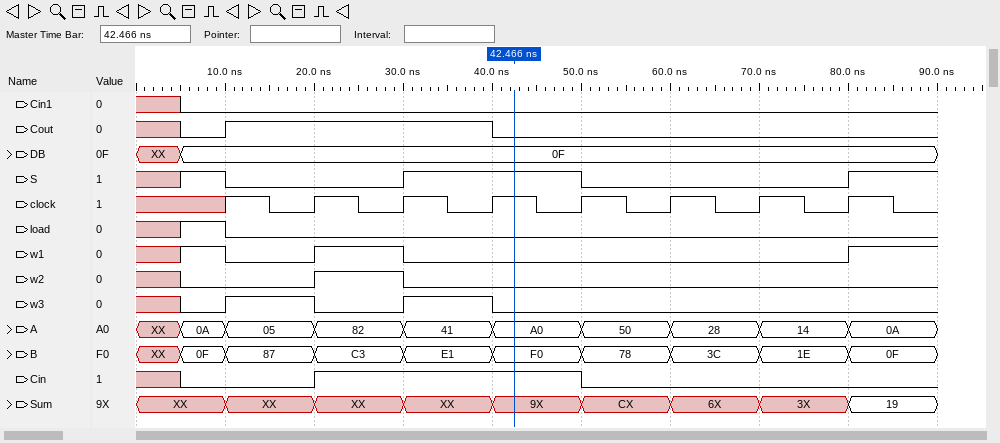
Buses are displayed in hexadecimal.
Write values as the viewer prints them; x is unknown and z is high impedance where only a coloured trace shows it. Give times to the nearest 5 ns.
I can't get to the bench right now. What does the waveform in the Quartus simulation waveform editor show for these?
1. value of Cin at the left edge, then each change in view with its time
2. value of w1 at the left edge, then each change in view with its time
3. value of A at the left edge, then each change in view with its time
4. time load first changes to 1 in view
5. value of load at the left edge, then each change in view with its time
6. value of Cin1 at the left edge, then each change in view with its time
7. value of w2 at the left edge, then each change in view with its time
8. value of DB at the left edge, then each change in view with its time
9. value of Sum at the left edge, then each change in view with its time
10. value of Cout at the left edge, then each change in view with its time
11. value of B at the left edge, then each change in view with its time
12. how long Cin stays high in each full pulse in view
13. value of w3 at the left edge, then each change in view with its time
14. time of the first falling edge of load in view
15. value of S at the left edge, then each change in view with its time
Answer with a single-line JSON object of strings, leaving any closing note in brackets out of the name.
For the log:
{"value of Cin at the left edge, then each change in view with its time": "x, 0 at 5 ns, 1 at 20 ns, 0 at 50 ns", "value of w1 at the left edge, then each change in view with its time": "x, 1 at 5 ns, 0 at 10 ns, 1 at 20 ns, 0 at 30 ns, 1 at 80 ns", "value of A at the left edge, then each change in view with its time": "XX, 0A at 5 ns, 05 at 10 ns, 82 at 20 ns, 41 at 30 ns, A0 at 40 ns, 50 at 50 ns, 28 at 60 ns, 14 at 70 ns, 0A at 80 ns", "time load first changes to 1 in view": "5 ns", "value of load at the left edge, then each change in view with its time": "x, 1 at 5 ns, 0 at 10 ns", "value of Cin1 at the left edge, then each change in view with its time": "x, 0 at 5 ns", "value of w2 at the left edge, then each change in view with its time": "x, 0 at 5 ns, 1 at 20 ns, 0 at 30 ns", "value of DB at the left edge, then each change in view with its time": "XX, 0F at 5 ns", "value of Sum at the left edge, then each change in view with its time": "XX, XX at 10 ns, XX at 20 ns, XX at 30 ns, 9X at 40 ns, CX at 50 ns, 6X at 60 ns, 3X at 70 ns, 19 at 80 ns", "value of Cout at the left edge, then each change in view with its time": "x, 0 at 5 ns, 1 at 10 ns, 0 at 40 ns", "value of B at the left edge, then each change in view with its time": "XX, 0F at 5 ns, 87 at 10 ns, C3 at 20 ns, E1 at 30 ns, F0 at 40 ns, 78 at 50 ns, 3C at 60 ns, 1E at 70 ns, 0F at 80 ns", "how long Cin stays high in each full pulse in view": "30 ns", "value of w3 at the left edge, then each change in view with its time": "x, 0 at 5 ns, 1 at 10 ns, 0 at 20 ns, 1 at 30 ns, 0 at 40 ns", "time of the first falling edge of load in view": "10 ns", "value of S at the left edge, then each change in view with its time": "x, 1 at 5 ns, 0 at 10 ns, 1 at 30 ns, 0 at 50 ns, 1 at 80 ns"}
